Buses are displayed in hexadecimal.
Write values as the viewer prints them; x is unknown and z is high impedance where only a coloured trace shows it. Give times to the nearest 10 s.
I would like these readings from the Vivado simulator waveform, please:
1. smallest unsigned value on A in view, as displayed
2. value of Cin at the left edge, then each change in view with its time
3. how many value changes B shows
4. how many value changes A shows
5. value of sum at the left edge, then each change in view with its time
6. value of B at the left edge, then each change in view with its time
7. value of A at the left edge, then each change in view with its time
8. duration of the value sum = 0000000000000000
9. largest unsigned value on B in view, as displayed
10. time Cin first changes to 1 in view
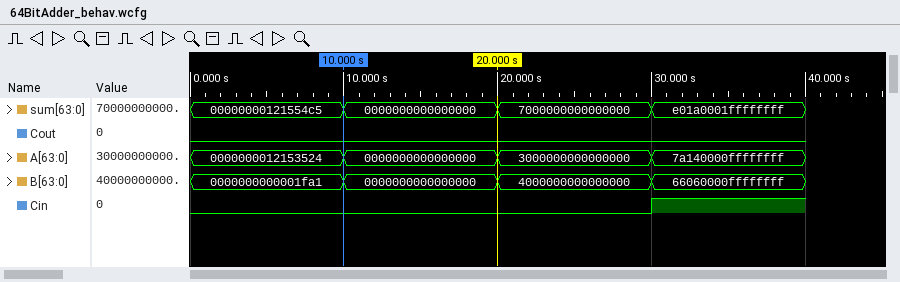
0000000000000000
0, 1 at 30 s
3
3
00000000121554c5, 0000000000000000 at 10 s, 7000000000000000 at 20 s, e01a0001ffffffff at 30 s
0000000000001fa1, 0000000000000000 at 10 s, 4000000000000000 at 20 s, 66060000ffffffff at 30 s
0000000012153524, 0000000000000000 at 10 s, 3000000000000000 at 20 s, 7a140000ffffffff at 30 s
10 s
66060000ffffffff
30 s
